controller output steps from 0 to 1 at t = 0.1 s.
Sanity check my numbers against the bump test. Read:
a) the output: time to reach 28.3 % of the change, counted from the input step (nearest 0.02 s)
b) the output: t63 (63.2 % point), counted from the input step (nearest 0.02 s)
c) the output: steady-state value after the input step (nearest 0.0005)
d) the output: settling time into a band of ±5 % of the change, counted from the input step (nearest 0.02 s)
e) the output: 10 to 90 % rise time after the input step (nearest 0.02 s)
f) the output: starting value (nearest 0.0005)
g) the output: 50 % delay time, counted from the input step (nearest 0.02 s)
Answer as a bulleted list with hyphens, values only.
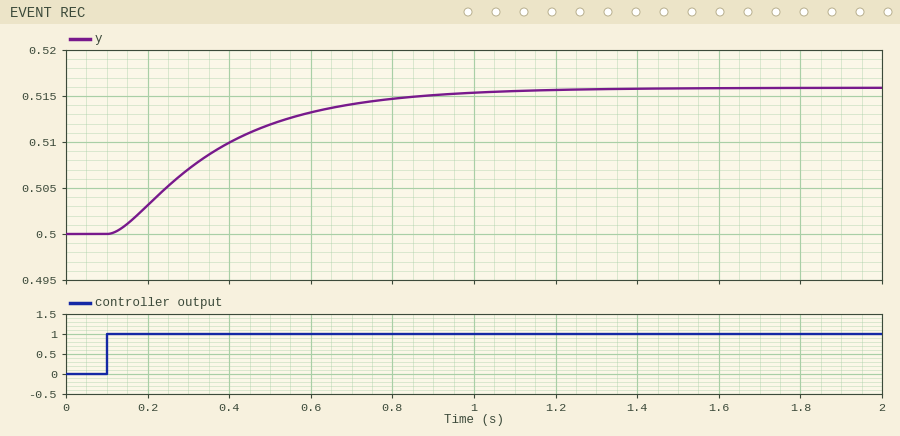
- 0.14 s
- 0.30 s
- 0.5160
- 0.80 s
- 0.56 s
- 0.5000
- 0.22 s
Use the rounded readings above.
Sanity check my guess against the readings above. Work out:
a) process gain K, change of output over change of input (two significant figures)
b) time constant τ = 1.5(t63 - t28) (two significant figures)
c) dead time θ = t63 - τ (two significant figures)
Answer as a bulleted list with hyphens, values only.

- 0.016
- 0.24 s
- 0.060 s
